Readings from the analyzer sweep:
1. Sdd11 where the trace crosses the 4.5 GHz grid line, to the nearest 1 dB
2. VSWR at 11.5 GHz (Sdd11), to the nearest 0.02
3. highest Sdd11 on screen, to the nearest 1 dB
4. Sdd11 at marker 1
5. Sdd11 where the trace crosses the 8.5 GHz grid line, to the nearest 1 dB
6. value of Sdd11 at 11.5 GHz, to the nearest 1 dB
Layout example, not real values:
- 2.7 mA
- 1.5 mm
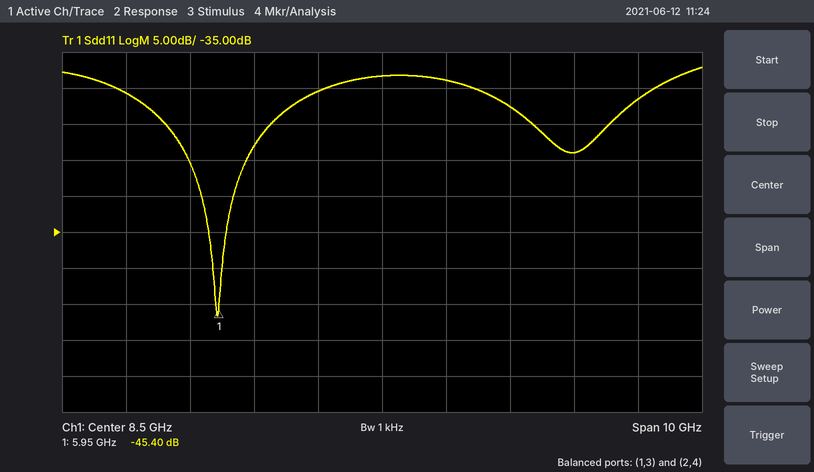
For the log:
- -16 dB
- 1.14
- -12 dB
- -45.40 dB
- -13 dB
- -24 dB
